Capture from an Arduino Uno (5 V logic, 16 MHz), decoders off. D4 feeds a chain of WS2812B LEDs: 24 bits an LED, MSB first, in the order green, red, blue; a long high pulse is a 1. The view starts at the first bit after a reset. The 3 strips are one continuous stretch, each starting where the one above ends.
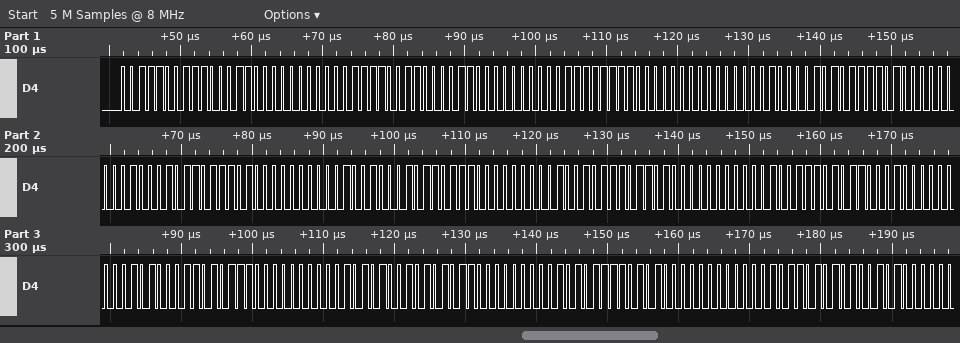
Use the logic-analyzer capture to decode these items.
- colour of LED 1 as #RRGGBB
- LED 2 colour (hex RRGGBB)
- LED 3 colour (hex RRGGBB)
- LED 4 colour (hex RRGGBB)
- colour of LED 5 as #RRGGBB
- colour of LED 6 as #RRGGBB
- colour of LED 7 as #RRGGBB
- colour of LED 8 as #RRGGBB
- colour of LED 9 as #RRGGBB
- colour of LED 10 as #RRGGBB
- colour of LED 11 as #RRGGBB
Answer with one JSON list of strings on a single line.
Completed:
["#C63900", "#C33C00", "#C03F00", "#BD4200", "#BA4500", "#B74800", "#B44B00", "#B14E00", "#AE5100", "#AB5400", "#A85700"]
